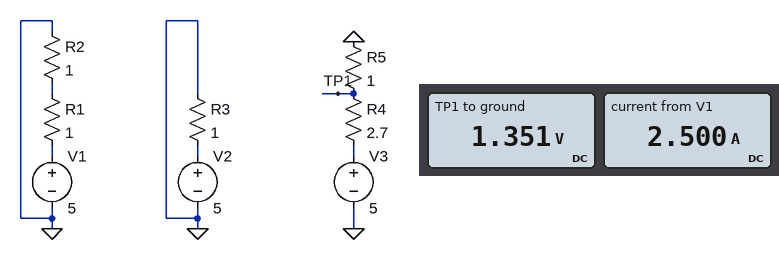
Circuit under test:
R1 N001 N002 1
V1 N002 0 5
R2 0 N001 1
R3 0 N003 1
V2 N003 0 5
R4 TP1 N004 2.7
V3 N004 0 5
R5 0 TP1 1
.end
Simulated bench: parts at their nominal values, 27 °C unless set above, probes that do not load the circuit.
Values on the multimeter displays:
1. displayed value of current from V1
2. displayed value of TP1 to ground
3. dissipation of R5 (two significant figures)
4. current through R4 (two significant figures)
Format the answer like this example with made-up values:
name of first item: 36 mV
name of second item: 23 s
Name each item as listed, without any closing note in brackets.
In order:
displayed value of current from V1: 2.500 A
displayed value of TP1 to ground: 1.351 V
dissipation of R5: 1.8 W
current through R4: 1.4 A
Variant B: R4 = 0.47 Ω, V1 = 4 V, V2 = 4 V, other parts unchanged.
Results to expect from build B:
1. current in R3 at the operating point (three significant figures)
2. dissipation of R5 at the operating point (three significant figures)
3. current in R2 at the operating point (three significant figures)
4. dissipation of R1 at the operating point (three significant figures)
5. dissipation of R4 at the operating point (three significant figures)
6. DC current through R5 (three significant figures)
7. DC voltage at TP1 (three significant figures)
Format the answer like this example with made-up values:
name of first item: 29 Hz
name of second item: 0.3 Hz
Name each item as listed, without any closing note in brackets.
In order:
current in R3 at the operating point: 4.00 A
dissipation of R5 at the operating point: 11.6 W
current in R2 at the operating point: 2.00 A
dissipation of R1 at the operating point: 4.00 W
dissipation of R4 at the operating point: 5.44 W
DC current through R5: 3.40 A
DC voltage at TP1: 3.40 V
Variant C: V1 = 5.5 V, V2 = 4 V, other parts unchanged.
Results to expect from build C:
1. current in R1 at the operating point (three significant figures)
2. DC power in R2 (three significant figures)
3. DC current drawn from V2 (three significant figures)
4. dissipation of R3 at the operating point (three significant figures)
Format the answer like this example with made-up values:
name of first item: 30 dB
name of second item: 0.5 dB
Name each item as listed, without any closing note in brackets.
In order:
current in R1 at the operating point: 2.75 A
DC power in R2: 7.56 W
DC current drawn from V2: 4.00 A
dissipation of R3 at the operating point: 16.0 W
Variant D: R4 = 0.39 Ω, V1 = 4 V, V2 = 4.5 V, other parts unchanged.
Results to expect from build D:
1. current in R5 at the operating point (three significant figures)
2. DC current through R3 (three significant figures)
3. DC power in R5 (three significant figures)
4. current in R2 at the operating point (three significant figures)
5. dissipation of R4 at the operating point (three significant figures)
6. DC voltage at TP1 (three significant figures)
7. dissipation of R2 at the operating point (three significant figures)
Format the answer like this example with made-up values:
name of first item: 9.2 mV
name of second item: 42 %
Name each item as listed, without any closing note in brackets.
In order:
current in R5 at the operating point: 3.60 A
DC current through R3: 4.50 A
DC power in R5: 12.9 W
current in R2 at the operating point: 2.00 A
dissipation of R4 at the operating point: 5.05 W
DC voltage at TP1: 3.60 V
dissipation of R2 at the operating point: 4.00 W
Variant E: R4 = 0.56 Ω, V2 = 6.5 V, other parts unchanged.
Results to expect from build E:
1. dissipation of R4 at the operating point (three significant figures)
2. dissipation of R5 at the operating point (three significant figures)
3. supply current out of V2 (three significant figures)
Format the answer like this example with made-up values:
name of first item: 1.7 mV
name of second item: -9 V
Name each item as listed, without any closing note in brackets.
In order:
dissipation of R4 at the operating point: 5.75 W
dissipation of R5 at the operating point: 10.3 W
supply current out of V2: 6.50 A
